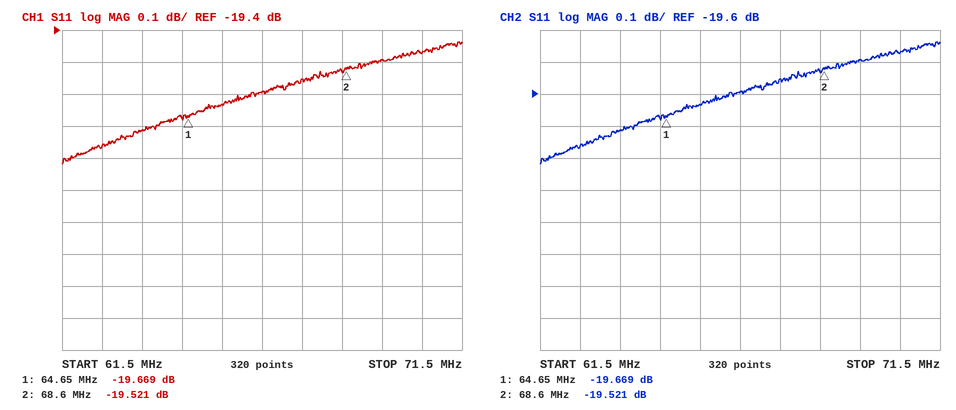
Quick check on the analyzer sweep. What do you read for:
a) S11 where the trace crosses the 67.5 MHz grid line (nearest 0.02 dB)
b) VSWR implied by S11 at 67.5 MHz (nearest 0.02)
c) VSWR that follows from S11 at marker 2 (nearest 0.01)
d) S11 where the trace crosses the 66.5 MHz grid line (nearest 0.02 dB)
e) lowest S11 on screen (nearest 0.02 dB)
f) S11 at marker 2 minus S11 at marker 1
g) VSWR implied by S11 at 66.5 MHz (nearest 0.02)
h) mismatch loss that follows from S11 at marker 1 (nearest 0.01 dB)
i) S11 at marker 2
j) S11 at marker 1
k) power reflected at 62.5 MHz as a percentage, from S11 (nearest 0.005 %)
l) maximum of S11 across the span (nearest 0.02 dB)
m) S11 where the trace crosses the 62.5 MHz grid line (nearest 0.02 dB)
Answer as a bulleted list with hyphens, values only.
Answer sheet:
- -19.56 dB
- 1.24
- 1.24
- -19.60 dB
- -19.82 dB
- 0.148 dB
- 1.24
- 0.05 dB
- -19.521 dB
- -19.669 dB
- 1.055 %
- -19.44 dB
- -19.76 dB
